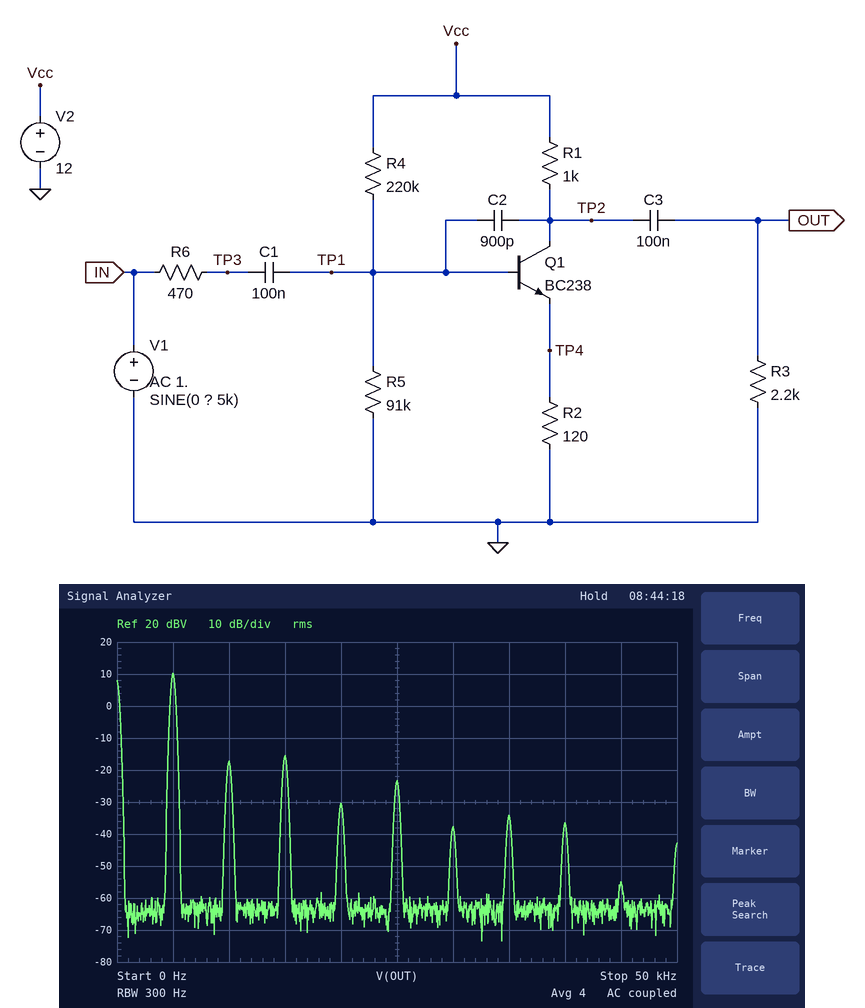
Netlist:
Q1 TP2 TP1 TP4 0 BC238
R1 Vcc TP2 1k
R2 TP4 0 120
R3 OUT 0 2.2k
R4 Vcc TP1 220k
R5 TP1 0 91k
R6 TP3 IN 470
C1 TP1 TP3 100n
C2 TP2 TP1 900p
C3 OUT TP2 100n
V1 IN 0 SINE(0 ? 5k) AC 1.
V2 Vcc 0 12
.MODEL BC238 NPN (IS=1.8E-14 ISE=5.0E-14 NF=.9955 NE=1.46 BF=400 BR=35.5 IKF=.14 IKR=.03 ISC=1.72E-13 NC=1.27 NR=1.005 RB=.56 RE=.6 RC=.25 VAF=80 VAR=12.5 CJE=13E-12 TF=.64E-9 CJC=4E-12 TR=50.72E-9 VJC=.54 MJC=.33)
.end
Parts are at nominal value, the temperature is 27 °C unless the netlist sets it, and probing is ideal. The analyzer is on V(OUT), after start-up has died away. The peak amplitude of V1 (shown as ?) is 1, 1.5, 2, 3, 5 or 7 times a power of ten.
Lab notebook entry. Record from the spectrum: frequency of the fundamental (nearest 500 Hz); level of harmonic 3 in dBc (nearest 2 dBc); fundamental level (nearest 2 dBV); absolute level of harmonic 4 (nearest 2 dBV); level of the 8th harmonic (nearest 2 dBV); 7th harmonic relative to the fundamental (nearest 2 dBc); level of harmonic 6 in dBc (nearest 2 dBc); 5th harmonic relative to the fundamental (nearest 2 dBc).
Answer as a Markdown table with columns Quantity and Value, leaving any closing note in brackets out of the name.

| Quantity | Value |
|---|---|
| frequency of the fundamental | 5.0 kHz |
| level of harmonic 3 in dBc | -26 dBc |
| fundamental level | 10 dBV |
| absolute level of harmonic 4 | -30 dBV |
| level of the 8th harmonic | -36 dBV |
| 7th harmonic relative to the fundamental | -44 dBc |
| level of harmonic 6 in dBc | -48 dBc |
| 5th harmonic relative to the fundamental | -34 dBc |
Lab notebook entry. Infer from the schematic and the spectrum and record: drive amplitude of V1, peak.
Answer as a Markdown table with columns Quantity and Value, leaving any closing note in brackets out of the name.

| Quantity | Value |
|---|---|
| drive amplitude of V1, peak | 1 V |
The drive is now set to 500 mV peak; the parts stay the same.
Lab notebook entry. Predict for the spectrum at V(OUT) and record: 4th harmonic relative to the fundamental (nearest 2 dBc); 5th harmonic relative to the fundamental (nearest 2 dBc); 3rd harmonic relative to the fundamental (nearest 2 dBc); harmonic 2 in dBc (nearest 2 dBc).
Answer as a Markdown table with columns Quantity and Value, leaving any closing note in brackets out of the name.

| Quantity | Value |
|---|---|
| 4th harmonic relative to the fundamental | -48 dBc |
| 5th harmonic relative to the fundamental | -50 dBc |
| 3rd harmonic relative to the fundamental | -46 dBc |
| harmonic 2 in dBc | -52 dBc |
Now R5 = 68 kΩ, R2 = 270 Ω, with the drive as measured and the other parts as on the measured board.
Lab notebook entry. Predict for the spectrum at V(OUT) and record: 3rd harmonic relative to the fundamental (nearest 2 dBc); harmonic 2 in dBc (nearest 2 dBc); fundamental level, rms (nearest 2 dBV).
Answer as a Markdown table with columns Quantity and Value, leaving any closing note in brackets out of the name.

| Quantity | Value |
|---|---|
| 3rd harmonic relative to the fundamental | -58 dBc |
| harmonic 2 in dBc | -48 dBc |
| fundamental level, rms | 4 dBV |
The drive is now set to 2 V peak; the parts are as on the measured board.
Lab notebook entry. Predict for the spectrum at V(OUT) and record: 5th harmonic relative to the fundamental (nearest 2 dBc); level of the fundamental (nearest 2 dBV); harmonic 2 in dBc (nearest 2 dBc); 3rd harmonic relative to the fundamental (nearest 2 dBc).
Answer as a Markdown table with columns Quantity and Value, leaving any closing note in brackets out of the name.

| Quantity | Value |
|---|---|
| 5th harmonic relative to the fundamental | -32 dBc |
| level of the fundamental | 10 dBV |
| harmonic 2 in dBc | -8 dBc |
| 3rd harmonic relative to the fundamental | -32 dBc |
